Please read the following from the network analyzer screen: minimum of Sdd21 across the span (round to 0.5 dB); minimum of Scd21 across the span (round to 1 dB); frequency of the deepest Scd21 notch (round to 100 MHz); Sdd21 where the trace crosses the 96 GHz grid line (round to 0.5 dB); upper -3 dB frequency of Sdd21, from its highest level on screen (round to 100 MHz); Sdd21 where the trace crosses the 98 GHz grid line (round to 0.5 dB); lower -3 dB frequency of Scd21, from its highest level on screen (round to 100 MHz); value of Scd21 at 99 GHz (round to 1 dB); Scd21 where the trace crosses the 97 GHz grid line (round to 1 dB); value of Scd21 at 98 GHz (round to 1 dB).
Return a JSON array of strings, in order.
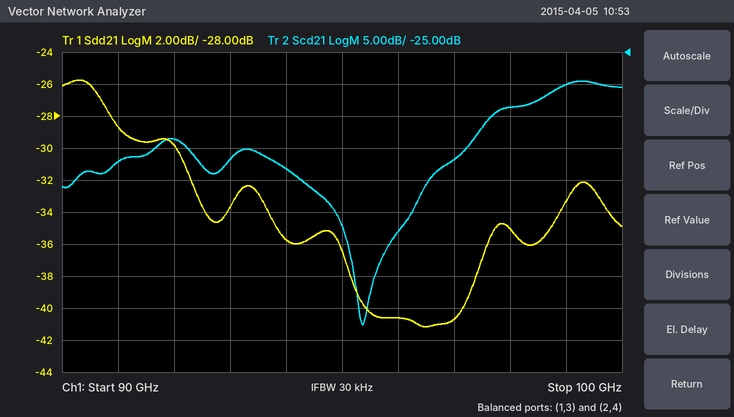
["-41.0 dB", "-68 dB", "95.4 GHz", "-40.5 dB", "91.0 GHz", "-35.0 dB", "98.5 GHz", "-30 dB", "-42 dB", "-34 dB"]
